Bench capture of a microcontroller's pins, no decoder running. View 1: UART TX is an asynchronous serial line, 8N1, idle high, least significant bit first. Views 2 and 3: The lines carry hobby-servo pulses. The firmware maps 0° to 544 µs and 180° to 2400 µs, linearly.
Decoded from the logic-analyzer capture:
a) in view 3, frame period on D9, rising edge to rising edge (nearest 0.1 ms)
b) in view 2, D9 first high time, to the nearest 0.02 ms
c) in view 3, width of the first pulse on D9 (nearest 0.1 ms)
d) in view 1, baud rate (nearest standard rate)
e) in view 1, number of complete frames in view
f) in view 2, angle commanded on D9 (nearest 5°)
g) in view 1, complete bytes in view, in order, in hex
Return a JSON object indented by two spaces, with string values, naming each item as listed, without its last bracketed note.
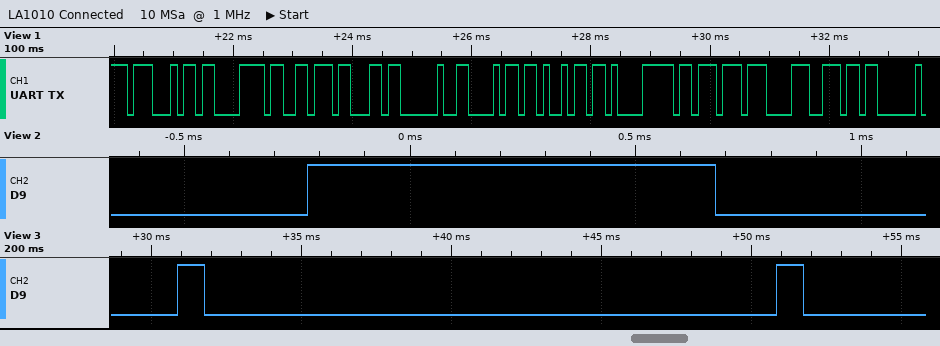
{
  "in view 3, frame period on D9, rising edge to rising edge": "20.0 ms",
  "in view 2, D9 first high time, to the nearest 0.02 ms": "0.90 ms",
  "in view 3, width of the first pulse on D9": "0.9 ms",
  "in view 1, baud rate": "9600 baud",
  "in view 1, number of complete frames in view": "11",
  "in view 2, angle commanded on D9": "35°",
  "in view 1, complete bytes in view, in order, in hex": "47 C3 B3 63 20 68 69 E1 BB 87 6E"
}
